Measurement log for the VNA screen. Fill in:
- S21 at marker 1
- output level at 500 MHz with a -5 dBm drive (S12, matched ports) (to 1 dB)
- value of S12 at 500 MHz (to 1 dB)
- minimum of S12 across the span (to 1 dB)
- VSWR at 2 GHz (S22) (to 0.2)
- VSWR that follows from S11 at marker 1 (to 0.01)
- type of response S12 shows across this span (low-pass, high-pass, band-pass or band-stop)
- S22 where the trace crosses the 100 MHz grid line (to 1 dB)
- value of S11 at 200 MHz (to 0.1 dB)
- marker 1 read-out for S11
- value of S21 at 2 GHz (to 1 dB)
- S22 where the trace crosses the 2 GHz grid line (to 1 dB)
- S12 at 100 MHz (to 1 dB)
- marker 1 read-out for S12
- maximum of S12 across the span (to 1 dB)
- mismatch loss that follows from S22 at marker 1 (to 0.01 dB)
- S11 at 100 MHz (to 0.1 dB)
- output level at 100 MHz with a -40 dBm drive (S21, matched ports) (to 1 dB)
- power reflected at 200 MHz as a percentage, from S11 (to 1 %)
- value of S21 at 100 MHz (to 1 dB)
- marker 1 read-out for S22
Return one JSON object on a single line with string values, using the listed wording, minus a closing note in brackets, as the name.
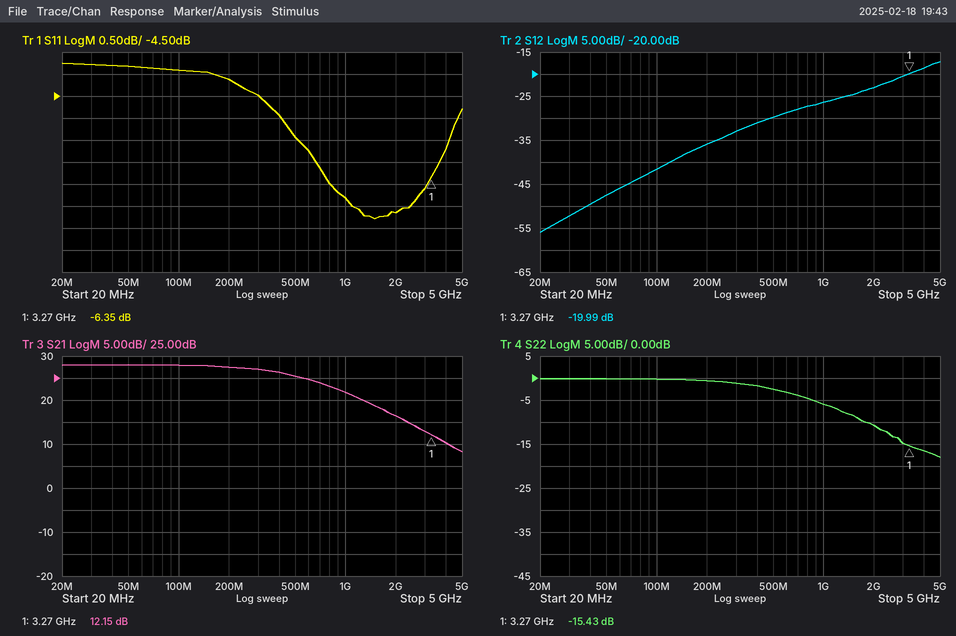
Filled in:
{"S21 at marker 1": "12.15 dB", "output level at 500 MHz with a -5 dBm drive (S12, matched ports)": "-35 dBm", "value of S12 at 500 MHz": "-30 dB", "minimum of S12 across the span": "-56 dB", "VSWR at 2 GHz (S22)": "1.8", "VSWR that follows from S11 at marker 1": "2.86", "type of response S12 shows across this span": "high-pass", "S22 where the trace crosses the 100 MHz grid line": "0 dB", "value of S11 at 200 MHz": "-4.1 dB", "marker 1 read-out for S11": "-6.35 dB", "value of S21 at 2 GHz": "16 dB", "S22 where the trace crosses the 2 GHz grid line": "-11 dB", "S12 at 100 MHz": "-42 dB", "marker 1 read-out for S12": "-19.99 dB", "maximum of S12 across the span": "-17 dB", "mismatch loss that follows from S22 at marker 1": "0.13 dB", "S11 at 100 MHz": "-3.9 dB", "output level at 100 MHz with a -40 dBm drive (S21, matched ports)": "-12 dBm", "power reflected at 200 MHz as a percentage, from S11": "39 %", "value of S21 at 100 MHz": "28 dB", "marker 1 read-out for S22": "-15.43 dB"}
